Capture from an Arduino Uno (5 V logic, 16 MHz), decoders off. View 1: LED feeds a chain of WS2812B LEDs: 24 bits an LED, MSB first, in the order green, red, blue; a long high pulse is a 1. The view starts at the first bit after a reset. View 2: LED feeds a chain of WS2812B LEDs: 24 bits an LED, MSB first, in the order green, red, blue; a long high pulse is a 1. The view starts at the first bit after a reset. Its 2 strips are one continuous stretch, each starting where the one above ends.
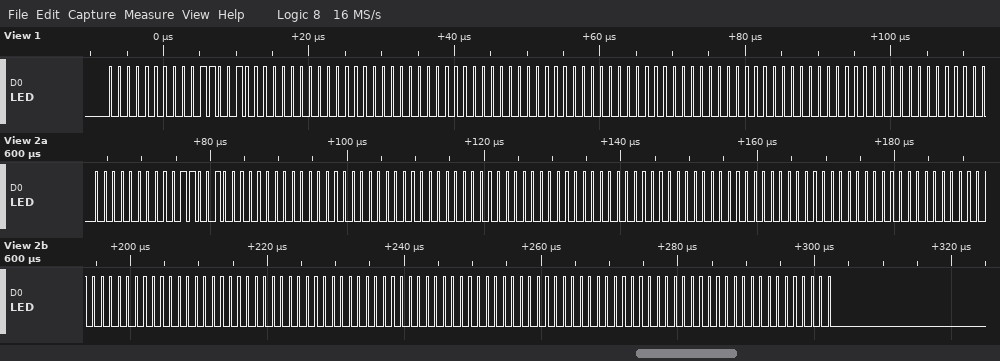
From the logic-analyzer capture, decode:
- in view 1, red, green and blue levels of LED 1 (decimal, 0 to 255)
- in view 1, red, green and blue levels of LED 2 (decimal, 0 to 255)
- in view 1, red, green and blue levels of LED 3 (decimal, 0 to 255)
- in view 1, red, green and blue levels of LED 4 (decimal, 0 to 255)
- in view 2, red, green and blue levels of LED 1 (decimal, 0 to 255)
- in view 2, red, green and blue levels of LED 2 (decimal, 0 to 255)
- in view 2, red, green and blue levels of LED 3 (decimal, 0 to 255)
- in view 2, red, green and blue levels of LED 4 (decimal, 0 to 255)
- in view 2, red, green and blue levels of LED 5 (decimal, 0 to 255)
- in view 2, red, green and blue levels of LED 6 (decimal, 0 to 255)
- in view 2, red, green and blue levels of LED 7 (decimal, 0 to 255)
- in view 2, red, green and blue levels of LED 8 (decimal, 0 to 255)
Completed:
50, 0, 0
0, 0, 0
0, 0, 0
0, 0, 0
50, 0, 0
0, 0, 0
0, 0, 0
0, 0, 0
0, 0, 0
0, 0, 0
0, 0, 0
0, 0, 0
